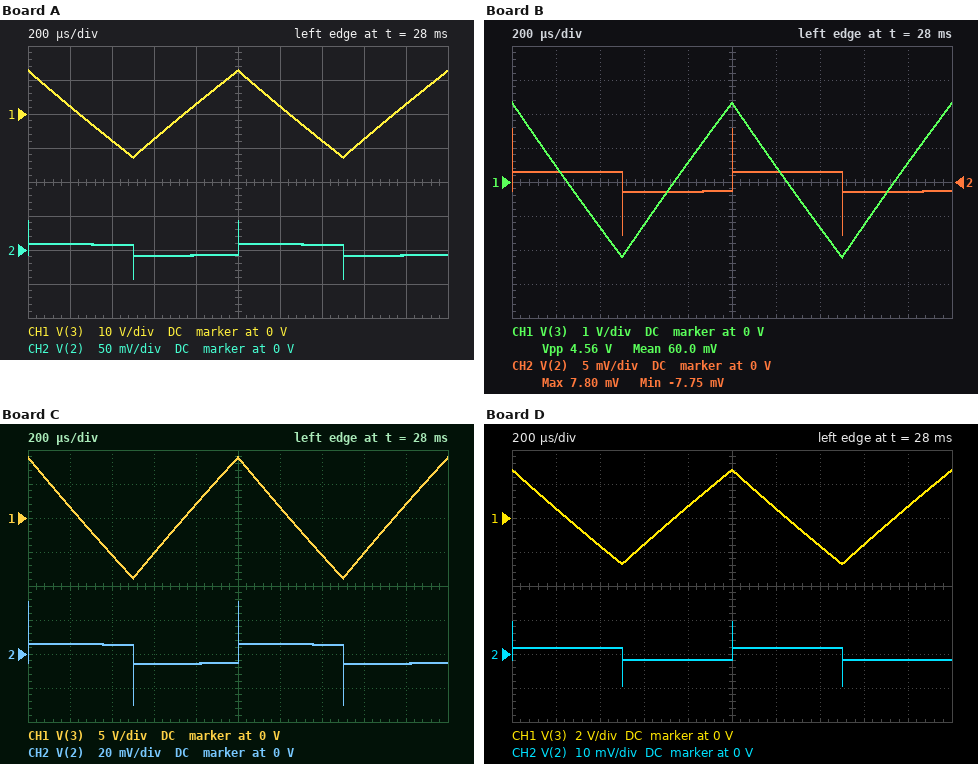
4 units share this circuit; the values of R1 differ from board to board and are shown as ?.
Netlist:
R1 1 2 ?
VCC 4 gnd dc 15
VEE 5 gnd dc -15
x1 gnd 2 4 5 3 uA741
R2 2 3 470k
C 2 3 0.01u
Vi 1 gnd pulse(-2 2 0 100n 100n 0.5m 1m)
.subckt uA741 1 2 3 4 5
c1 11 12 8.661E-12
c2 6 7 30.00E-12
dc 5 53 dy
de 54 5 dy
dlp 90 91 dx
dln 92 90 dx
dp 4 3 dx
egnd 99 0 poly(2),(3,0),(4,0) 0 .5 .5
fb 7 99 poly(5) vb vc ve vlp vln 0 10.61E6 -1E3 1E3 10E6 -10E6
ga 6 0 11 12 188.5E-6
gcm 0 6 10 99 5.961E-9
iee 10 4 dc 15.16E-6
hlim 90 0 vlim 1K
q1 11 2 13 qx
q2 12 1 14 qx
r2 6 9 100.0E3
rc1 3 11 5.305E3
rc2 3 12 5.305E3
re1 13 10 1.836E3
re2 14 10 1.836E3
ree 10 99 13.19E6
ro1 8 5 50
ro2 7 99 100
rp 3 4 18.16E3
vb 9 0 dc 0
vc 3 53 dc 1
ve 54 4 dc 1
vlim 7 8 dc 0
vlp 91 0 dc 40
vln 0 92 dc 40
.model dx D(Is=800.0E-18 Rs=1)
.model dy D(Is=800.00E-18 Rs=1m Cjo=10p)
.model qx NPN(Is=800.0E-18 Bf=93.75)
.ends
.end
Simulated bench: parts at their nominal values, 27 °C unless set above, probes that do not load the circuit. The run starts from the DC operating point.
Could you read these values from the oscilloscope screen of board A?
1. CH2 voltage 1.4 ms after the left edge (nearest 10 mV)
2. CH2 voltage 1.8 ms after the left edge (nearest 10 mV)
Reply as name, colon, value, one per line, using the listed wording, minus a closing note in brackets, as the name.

CH2 voltage 1.4 ms after the left edge: 10 mV
CH2 voltage 1.8 ms after the left edge: -10 mV
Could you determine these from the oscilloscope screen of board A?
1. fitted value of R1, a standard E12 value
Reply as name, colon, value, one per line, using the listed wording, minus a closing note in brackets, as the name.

fitted value of R1, a standard E12 value: 3.9 kΩ
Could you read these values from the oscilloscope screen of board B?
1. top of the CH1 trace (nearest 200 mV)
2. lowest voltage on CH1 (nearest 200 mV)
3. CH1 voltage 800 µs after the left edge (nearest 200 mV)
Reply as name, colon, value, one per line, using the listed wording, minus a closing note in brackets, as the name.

top of the CH1 trace: 2.4 V
lowest voltage on CH1: -2.2 V
CH1 voltage 800 µs after the left edge: 600 mV
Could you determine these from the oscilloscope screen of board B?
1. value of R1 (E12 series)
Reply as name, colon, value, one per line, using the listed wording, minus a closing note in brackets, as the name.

value of R1: 22 kΩ
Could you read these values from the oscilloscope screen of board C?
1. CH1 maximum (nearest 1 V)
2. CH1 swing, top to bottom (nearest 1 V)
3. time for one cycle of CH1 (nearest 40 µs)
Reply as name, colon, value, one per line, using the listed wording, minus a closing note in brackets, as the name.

CH1 maximum: 9 V
CH1 swing, top to bottom: 18 V
time for one cycle of CH1: 1.00 ms
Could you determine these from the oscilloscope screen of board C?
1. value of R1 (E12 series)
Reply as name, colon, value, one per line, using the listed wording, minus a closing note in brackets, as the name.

value of R1: 5.6 kΩ
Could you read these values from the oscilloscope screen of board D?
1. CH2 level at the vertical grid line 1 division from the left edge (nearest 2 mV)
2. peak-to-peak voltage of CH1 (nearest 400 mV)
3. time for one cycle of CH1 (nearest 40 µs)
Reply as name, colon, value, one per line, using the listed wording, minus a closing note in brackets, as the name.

CH2 level at the vertical grid line 1 division from the left edge: 2 mV
peak-to-peak voltage of CH1: 5.6 V
time for one cycle of CH1: 1.00 ms
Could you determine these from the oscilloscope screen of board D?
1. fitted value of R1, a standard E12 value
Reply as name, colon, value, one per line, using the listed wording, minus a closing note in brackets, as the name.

fitted value of R1, a standard E12 value: 18 kΩ
